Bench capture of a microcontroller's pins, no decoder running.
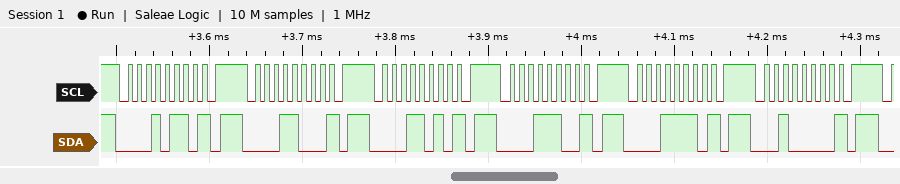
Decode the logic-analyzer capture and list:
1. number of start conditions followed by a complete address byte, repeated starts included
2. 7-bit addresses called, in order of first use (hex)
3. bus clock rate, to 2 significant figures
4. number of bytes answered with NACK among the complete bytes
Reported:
6
0x0B 0x0C 0x0D 0x0E 0x0F 0x10
100 kHz
6
